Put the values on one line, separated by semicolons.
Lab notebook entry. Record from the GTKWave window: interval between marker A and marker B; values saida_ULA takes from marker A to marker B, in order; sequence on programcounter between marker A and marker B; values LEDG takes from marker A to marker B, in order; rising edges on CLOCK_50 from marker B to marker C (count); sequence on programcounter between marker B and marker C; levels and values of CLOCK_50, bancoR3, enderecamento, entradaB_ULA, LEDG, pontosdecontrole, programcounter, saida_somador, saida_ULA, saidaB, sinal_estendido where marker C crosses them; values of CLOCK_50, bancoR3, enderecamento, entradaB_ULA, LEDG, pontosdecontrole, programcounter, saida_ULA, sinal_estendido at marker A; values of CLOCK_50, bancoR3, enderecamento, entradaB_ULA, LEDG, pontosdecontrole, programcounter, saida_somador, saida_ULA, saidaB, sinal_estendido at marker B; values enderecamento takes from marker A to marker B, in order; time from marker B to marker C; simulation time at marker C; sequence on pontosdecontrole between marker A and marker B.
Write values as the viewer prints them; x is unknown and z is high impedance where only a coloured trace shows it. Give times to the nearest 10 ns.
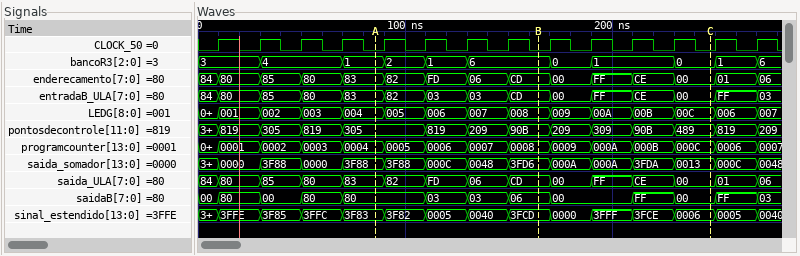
80 ns; 83, 82, FD, 06, CD; 0004, 0005, 0006, 0007, 0008; 004, 005, 006, 007, 008; 4; 0008, 0009, 000A, 000B, 000C; CLOCK_50=0, bancoR3=0, enderecamento=00, entradaB_ULA=00, LEDG=00C, pontosdecontrole=489, programcounter=000C, saida_somador=0013, saida_ULA=00, saidaB=00, sinal_estendido=0006; CLOCK_50=0, bancoR3=1, enderecamento=83, entradaB_ULA=83, LEDG=004, pontosdecontrole=305, programcounter=0004, saida_ULA=83, sinal_estendido=3F83; CLOCK_50=0, bancoR3=6, enderecamento=CD, entradaB_ULA=CD, LEDG=008, pontosdecontrole=90B, programcounter=0008, saida_somador=3FD6, saida_ULA=CD, saidaB=06, sinal_estendido=3FCD; 83, 82, FD, 06, CD; 80 ns; 250 ns; 305, 819, 209, 90B
